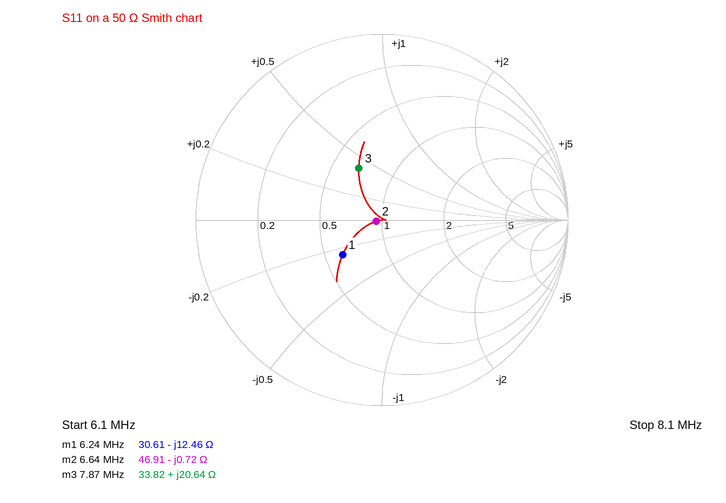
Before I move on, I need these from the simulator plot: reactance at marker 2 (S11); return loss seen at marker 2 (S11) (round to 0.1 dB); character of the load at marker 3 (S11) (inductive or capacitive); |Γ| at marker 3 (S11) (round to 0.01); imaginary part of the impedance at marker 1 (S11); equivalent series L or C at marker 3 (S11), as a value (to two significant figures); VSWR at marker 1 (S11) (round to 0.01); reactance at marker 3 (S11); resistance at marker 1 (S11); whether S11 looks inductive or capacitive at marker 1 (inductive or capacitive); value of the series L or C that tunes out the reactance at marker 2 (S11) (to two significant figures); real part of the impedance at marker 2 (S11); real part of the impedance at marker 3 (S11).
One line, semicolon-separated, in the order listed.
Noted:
-0.72 Ω; 29.7 dB; inductive; 0.30; -12.46 Ω; 420 nH; 1.79; +20.64 Ω; 30.61 Ω; capacitive; 17 nH; 46.91 Ω; 33.82 Ω
